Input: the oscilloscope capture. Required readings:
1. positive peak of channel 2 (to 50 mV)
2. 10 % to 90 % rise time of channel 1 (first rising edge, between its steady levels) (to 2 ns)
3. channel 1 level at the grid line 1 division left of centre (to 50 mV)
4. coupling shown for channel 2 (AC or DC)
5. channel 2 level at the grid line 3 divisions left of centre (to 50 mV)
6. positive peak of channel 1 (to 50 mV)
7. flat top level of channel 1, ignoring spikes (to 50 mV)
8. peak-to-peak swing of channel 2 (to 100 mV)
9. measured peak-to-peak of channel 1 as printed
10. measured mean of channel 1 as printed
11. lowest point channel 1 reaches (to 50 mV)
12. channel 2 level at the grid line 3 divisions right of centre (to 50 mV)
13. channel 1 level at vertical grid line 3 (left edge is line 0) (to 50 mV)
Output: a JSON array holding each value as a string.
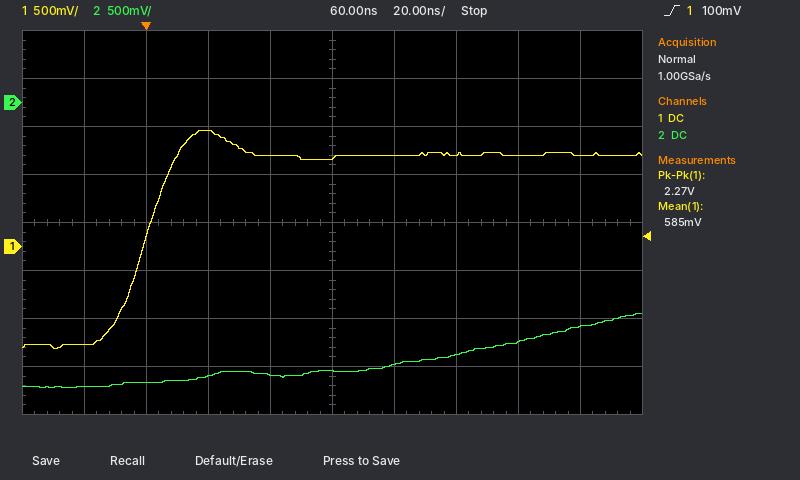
["-2.20 V", "18 ns", "950 mV", "DC", "-2.90 V", "1.20 V", "950 mV", "800 mV", "2.27 V", "585 mV", "-1.05 V", "-2.50 V", "1.20 V"]
